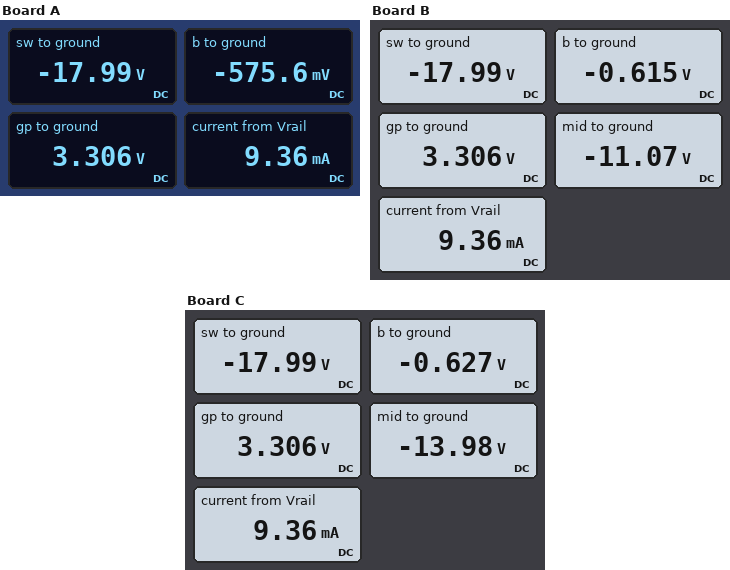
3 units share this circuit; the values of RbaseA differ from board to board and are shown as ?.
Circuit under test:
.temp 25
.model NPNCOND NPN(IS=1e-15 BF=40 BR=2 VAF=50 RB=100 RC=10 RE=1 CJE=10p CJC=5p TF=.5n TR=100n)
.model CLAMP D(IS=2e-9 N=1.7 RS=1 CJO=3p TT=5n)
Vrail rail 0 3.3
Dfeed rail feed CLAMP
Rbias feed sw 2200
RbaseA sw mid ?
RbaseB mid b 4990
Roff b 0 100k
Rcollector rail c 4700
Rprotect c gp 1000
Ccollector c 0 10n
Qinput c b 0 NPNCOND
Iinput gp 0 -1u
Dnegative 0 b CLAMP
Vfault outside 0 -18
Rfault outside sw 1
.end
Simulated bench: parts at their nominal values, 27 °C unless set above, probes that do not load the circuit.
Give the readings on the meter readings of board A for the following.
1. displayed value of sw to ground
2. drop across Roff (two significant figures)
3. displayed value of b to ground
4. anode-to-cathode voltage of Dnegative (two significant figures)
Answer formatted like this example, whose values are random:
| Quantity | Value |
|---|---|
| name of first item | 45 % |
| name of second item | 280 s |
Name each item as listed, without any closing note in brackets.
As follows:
| Quantity | Value |
|---|---|
| displayed value of sw to ground | -17.99 V |
| drop across Roff | 580 mV |
| displayed value of b to ground | -575.6 mV |
| anode-to-cathode voltage of Dnegative | 580 mV |
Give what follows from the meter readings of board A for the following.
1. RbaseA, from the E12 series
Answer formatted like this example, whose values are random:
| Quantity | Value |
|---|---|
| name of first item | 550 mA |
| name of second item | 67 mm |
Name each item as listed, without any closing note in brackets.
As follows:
| Quantity | Value |
|---|---|
| RbaseA, from the E12 series | 15 kΩ |
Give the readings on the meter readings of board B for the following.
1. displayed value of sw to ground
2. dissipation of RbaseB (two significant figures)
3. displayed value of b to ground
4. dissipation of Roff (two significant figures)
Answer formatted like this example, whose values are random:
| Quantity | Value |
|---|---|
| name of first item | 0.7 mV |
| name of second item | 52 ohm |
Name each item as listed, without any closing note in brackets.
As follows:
| Quantity | Value |
|---|---|
| displayed value of sw to ground | -17.99 V |
| dissipation of RbaseB | 22 mW |
| displayed value of b to ground | -0.615 V |
| dissipation of Roff | 3.8 µW |
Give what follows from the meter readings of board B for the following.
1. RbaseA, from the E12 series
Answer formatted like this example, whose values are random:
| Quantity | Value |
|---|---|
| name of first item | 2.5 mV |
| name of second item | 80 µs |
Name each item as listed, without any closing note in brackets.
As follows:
| Quantity | Value |
|---|---|
| RbaseA, from the E12 series | 3.3 kΩ |
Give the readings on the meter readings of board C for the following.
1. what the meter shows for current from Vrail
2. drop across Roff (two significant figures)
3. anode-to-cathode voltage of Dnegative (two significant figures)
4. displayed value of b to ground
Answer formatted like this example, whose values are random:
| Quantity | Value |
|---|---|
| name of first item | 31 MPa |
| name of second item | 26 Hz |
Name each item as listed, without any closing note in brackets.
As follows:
| Quantity | Value |
|---|---|
| what the meter shows for current from Vrail | 9.36 mA |
| drop across Roff | 630 mV |
| anode-to-cathode voltage of Dnegative | 630 mV |
| displayed value of b to ground | -0.627 V |
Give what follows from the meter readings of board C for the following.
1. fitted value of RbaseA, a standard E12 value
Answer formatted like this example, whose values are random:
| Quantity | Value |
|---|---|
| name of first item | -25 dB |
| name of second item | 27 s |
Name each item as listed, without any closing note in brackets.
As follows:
| Quantity | Value |
|---|---|
| fitted value of RbaseA, a standard E12 value | 1.5 kΩ |
